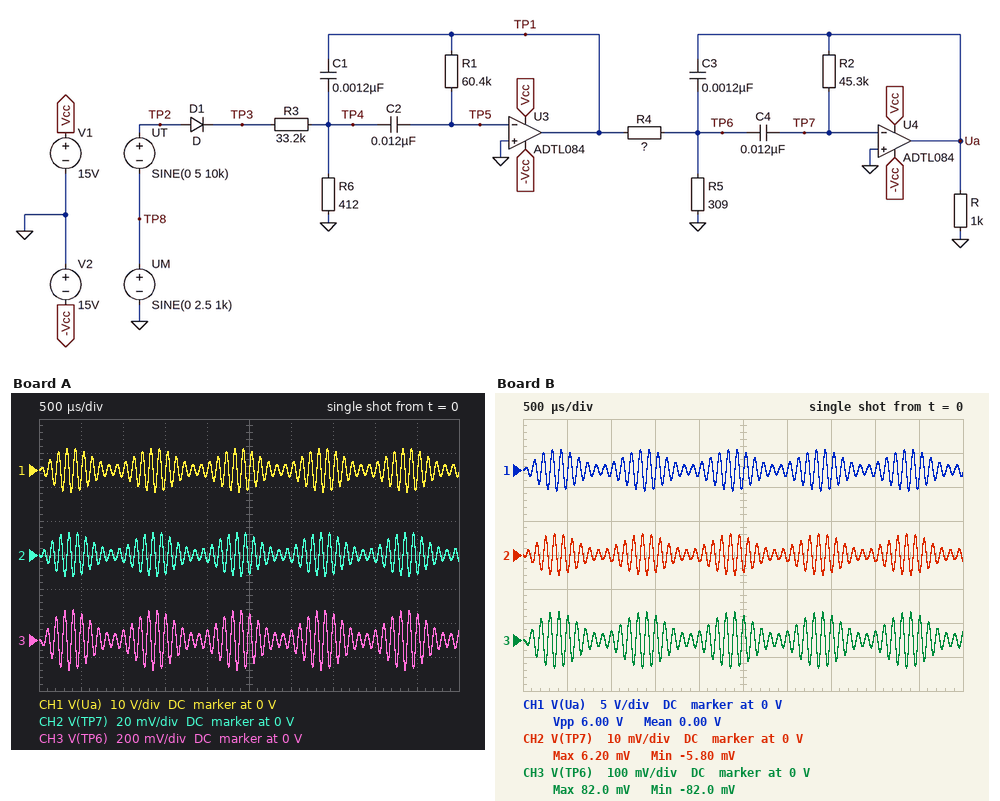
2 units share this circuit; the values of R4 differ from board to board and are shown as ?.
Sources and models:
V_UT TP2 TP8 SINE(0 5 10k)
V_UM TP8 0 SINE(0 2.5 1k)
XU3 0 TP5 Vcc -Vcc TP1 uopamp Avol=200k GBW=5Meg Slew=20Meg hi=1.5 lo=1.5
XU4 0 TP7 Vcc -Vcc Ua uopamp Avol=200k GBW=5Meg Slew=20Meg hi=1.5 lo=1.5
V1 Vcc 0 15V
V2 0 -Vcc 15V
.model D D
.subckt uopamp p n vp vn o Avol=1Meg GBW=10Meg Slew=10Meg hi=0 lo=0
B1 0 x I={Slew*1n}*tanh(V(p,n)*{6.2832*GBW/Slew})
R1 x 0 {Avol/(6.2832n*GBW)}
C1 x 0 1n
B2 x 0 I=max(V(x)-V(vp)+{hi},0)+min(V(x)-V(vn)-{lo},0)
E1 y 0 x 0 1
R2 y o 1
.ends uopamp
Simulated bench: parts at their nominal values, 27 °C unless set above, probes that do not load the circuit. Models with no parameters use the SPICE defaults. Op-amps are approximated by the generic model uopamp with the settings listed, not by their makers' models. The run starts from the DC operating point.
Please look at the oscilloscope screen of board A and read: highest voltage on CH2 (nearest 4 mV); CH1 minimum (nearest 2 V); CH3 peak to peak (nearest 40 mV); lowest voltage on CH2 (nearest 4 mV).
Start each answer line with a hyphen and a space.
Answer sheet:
- 12 mV
- -6 V
- 360 mV
- -12 mV
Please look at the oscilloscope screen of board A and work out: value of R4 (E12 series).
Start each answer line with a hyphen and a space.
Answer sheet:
- 18 kΩ
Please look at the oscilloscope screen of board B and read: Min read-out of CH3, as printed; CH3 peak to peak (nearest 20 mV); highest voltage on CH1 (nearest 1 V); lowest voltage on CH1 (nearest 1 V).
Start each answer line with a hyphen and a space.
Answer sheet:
- -82.0 mV
- 160 mV
- 3 V
- -3 V
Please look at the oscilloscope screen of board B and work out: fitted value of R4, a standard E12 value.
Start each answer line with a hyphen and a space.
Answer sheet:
- 39 kΩ
